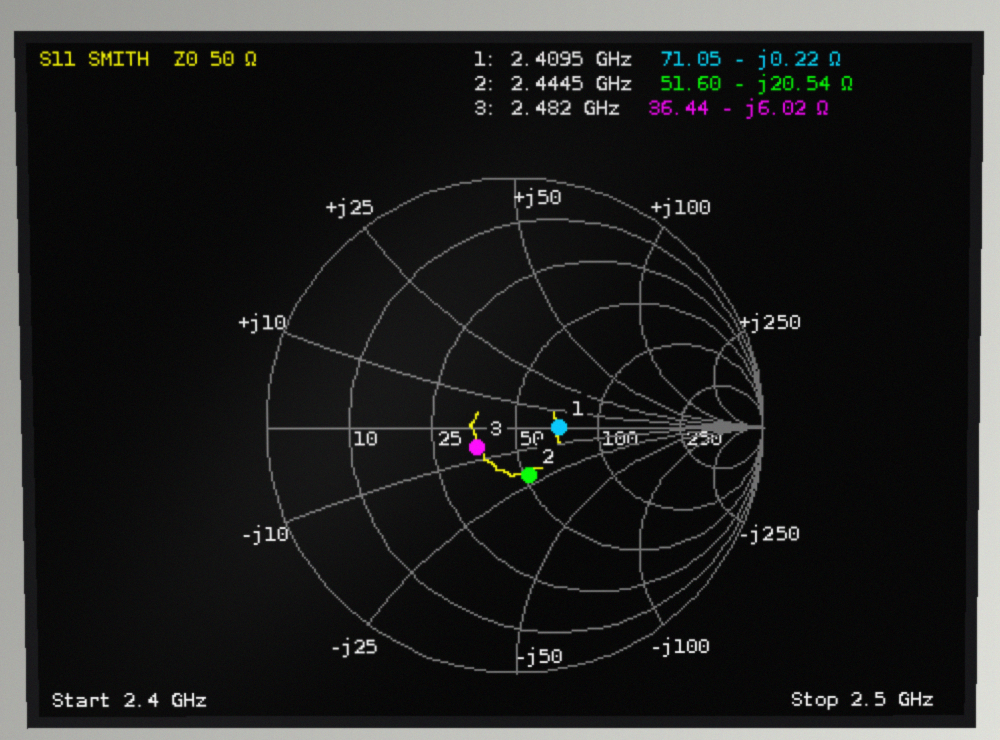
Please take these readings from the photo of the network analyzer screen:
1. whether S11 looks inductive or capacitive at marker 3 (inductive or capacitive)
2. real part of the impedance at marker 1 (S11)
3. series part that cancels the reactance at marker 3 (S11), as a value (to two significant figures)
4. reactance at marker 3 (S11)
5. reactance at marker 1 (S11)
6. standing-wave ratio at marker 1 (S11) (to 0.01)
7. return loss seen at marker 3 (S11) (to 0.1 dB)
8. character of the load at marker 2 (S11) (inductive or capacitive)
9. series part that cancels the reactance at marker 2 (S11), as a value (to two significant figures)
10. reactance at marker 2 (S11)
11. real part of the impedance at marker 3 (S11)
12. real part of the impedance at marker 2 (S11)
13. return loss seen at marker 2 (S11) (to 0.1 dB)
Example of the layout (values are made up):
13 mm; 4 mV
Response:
capacitive; 71.05 Ω; 390 pH; -6.02 Ω; -0.22 Ω; 1.42; 15.3 dB; capacitive; 1.3 nH; -20.54 Ω; 36.44 Ω; 51.60 Ω; 14.0 dB
